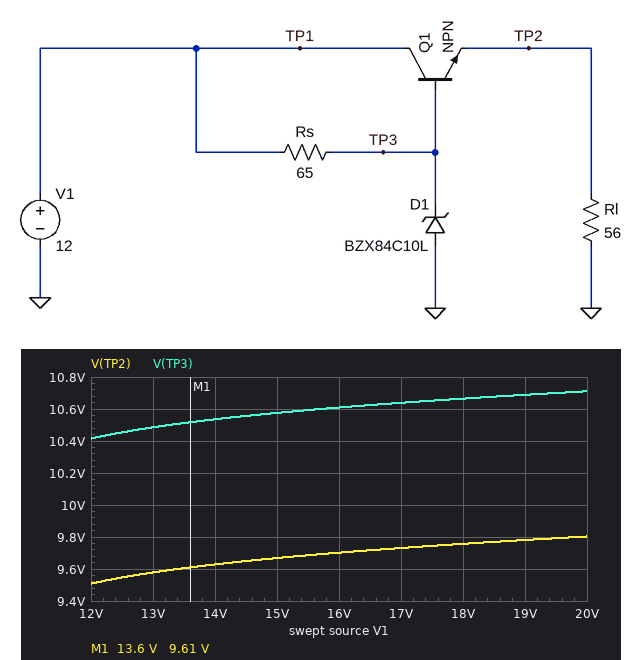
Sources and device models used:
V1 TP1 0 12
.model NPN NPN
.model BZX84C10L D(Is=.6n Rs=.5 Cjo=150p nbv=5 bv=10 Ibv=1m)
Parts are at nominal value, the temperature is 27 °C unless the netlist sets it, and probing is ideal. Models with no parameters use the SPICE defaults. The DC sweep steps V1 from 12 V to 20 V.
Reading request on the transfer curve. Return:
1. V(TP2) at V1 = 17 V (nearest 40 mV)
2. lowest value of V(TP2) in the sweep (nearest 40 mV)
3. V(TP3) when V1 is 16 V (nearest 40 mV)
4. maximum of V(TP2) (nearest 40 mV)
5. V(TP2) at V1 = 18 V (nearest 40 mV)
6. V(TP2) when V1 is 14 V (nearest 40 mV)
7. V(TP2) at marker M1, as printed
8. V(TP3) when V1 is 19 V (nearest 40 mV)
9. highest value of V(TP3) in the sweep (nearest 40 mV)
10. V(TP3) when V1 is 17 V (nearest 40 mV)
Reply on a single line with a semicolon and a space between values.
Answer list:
9.72 V; 9.52 V; 10.60 V; 9.80 V; 9.76 V; 9.64 V; 9.61 V; 10.68 V; 10.72 V; 10.64 V
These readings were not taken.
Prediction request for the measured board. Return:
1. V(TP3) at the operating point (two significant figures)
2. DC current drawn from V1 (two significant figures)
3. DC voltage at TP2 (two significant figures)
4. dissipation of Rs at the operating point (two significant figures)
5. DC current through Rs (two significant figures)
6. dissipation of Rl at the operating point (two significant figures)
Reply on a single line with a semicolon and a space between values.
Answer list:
10 V; 190 mA; 9.5 V; 39 mW; 24 mA; 1.6 W
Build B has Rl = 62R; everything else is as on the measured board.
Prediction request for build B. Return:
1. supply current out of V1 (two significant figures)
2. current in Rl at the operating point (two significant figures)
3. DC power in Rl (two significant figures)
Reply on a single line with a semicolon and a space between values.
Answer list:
180 mA; 150 mA; 1.5 W
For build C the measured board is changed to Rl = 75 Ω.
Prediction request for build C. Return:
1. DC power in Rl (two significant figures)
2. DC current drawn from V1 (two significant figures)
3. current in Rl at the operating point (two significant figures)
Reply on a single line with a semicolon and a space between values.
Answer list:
1.2 W; 150 mA; 130 mA
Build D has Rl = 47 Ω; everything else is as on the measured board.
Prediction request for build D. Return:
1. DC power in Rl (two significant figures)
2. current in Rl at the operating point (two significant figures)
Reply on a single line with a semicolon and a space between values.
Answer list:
1.9 W; 200 mA
